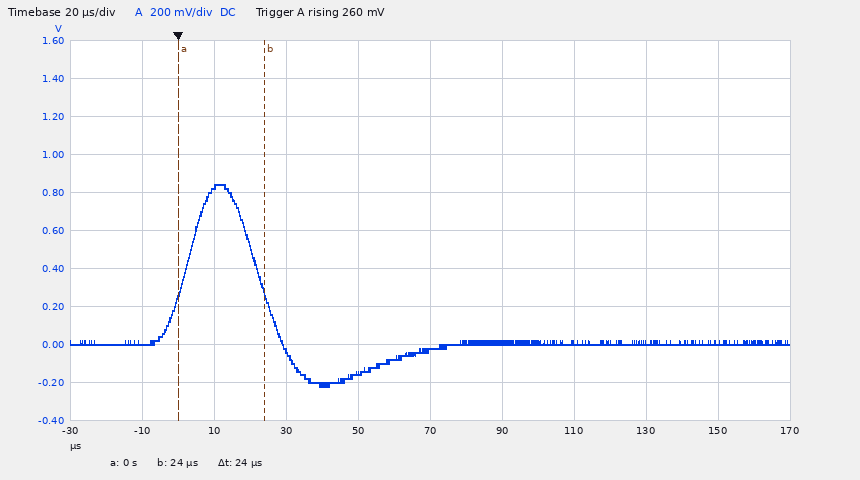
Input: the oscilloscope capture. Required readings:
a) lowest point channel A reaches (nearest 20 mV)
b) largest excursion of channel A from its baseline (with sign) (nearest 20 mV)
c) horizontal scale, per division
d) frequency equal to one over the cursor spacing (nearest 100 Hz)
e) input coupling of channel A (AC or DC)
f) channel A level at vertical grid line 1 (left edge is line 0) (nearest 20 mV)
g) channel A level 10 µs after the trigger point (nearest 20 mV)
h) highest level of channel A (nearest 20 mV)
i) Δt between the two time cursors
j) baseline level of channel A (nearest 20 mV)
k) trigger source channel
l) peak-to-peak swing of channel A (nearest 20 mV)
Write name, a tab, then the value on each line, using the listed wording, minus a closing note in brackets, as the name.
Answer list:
lowest point channel A reaches	-220 mV
largest excursion of channel A from its baseline (with sign)	+840 mV
horizontal scale, per division	20 µs
frequency equal to one over the cursor spacing	41.7 kHz
input coupling of channel A	DC
channel A level at vertical grid line 1 (left edge is line 0)	0 mV
channel A level 10 µs after the trigger point	820 mV
highest level of channel A	840 mV
Δt between the two time cursors	24 µs
baseline level of channel A	0 mV
trigger source channel	channel A
peak-to-peak swing of channel A	1.06 V
